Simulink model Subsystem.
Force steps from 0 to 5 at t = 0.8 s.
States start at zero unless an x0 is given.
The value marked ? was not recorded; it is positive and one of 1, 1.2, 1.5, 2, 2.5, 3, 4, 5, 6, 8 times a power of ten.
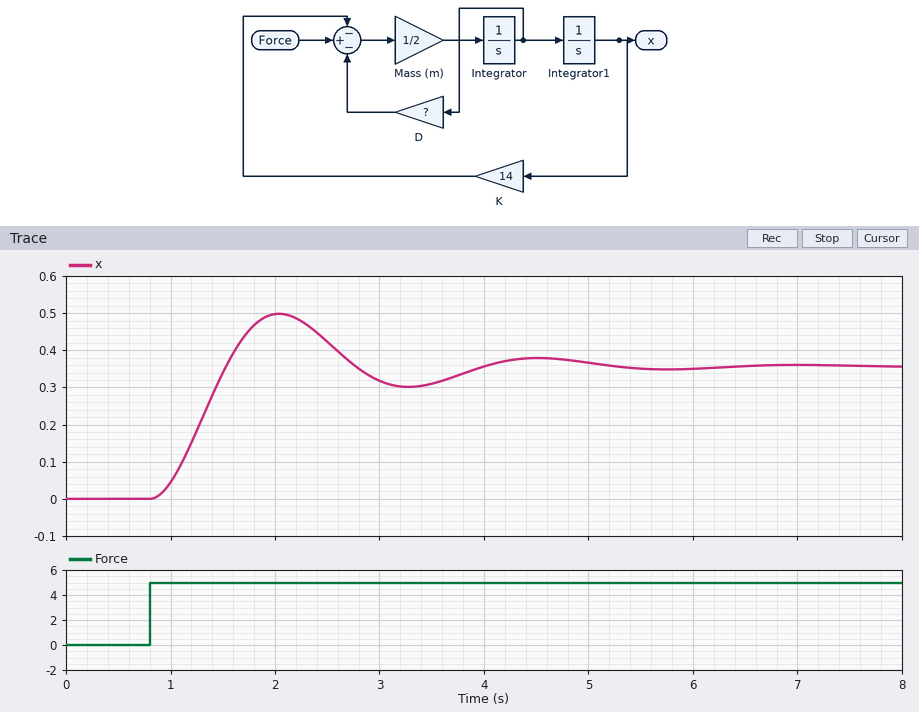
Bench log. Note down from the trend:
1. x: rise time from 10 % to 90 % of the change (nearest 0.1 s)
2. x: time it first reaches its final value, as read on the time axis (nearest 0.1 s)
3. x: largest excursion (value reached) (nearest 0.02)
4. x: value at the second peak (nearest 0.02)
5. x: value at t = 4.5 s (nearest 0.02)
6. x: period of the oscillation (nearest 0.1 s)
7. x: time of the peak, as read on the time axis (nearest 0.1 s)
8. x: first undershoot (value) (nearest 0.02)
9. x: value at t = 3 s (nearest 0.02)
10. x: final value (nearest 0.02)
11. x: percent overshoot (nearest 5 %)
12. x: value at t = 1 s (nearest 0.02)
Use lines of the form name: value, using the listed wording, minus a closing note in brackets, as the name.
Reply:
x: rise time from 10 % to 90 % of the change: 0.5 s
x: time it first reaches its final value, as read on the time axis: 1.5 s
x: largest excursion (value reached): 0.50
x: value at the second peak: 0.38
x: value at t = 4.5 s: 0.38
x: period of the oscillation: 2.5 s
x: time of the peak, as read on the time axis: 2.0 s
x: first undershoot (value): 0.30
x: value at t = 3 s: 0.32
x: final value: 0.36
x: percent overshoot: 40 %
x: value at t = 1 s: 0.04
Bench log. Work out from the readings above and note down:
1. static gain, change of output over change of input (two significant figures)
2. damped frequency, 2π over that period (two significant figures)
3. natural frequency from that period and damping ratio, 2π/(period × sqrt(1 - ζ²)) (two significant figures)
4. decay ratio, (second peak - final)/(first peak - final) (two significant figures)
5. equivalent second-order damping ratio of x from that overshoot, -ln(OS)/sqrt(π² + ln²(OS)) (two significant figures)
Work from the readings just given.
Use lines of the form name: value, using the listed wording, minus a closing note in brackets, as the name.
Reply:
static gain, change of output over change of input: 0.072
damped frequency, 2π over that period: 2.5 rad/s
natural frequency from that period and damping ratio, 2π/(period × sqrt(1 - ζ²)): 2.6 rad/s
decay ratio, (second peak - final)/(first peak - final): 0.14
equivalent second-order damping ratio of x from that overshoot, -ln(OS)/sqrt(π² + ln²(OS)): 0.28
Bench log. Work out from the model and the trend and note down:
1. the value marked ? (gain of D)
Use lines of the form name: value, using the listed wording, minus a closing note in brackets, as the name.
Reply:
the value marked ?: 3
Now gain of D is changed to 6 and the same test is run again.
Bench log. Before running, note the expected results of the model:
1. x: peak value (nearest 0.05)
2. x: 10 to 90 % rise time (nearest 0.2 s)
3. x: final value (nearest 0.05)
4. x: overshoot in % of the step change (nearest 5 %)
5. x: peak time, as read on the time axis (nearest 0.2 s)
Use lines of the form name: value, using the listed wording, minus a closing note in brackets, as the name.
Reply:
x: peak value: 0.40
x: 10 to 90 % rise time: 0.6 s
x: final value: 0.35
x: overshoot in % of the step change: 10 %
x: peak time, as read on the time axis: 2.2 s
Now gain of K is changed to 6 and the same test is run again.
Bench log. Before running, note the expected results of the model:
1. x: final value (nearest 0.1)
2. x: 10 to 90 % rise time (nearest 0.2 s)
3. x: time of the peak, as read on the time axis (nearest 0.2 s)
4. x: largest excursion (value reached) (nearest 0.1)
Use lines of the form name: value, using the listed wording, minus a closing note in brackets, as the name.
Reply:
x: final value: 0.8
x: 10 to 90 % rise time: 0.8 s
x: time of the peak, as read on the time axis: 2.8 s
x: largest excursion (value reached): 1.0
